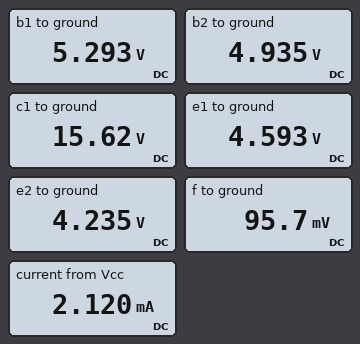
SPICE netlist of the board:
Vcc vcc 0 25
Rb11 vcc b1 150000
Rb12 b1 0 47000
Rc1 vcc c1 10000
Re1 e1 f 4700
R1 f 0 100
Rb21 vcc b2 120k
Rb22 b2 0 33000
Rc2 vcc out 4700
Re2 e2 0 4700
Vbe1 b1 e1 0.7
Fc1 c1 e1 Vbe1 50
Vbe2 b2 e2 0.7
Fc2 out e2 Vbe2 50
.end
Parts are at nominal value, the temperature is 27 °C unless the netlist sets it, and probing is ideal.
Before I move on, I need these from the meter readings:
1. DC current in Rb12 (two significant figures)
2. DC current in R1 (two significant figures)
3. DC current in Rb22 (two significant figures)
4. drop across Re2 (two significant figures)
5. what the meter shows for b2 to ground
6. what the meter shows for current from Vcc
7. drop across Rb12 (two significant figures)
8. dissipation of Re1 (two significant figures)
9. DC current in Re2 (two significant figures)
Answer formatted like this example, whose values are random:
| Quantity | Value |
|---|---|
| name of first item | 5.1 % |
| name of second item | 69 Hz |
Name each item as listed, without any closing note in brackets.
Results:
| Quantity | Value |
|---|---|
| DC current in Rb12 | 110 µA |
| DC current in R1 | 960 µA |
| DC current in Rb22 | 150 µA |
| drop across Re2 | 4.2 V |
| what the meter shows for b2 to ground | 4.935 V |
| what the meter shows for current from Vcc | 2.120 mA |
| drop across Rb12 | 5.3 V |
| dissipation of Re1 | 4.3 mW |
| DC current in Re2 | 900 µA |
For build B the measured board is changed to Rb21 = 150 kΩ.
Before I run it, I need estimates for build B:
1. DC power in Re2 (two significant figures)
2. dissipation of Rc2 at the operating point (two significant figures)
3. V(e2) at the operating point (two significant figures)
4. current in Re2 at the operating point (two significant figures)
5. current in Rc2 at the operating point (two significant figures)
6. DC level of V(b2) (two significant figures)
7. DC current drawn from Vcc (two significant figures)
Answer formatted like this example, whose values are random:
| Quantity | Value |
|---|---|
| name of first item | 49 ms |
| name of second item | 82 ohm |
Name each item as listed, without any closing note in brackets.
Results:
| Quantity | Value |
|---|---|
| DC power in Re2 | 2.5 mW |
| dissipation of Rc2 at the operating point | 2.4 mW |
| V(e2) at the operating point | 3.4 V |
| current in Re2 at the operating point | 730 µA |
| current in Rc2 at the operating point | 710 µA |
| DC level of V(b2) | 4.1 V |
| DC current drawn from Vcc | 1.9 mA |
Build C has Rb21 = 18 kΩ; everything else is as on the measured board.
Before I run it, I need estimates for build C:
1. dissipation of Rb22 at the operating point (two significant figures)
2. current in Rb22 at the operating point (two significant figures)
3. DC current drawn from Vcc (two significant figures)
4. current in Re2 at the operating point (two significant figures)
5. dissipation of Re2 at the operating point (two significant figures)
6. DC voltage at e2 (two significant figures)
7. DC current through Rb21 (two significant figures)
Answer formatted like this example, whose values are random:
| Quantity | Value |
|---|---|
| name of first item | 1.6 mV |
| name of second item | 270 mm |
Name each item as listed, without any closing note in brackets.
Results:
| Quantity | Value |
|---|---|
| dissipation of Rb22 at the operating point | 7.2 mW |
| current in Rb22 at the operating point | 470 µA |
| DC current drawn from Vcc | 4.7 mA |
| current in Re2 at the operating point | 3.1 mA |
| dissipation of Re2 at the operating point | 46 mW |
| DC voltage at e2 | 15 V |
| DC current through Rb21 | 530 µA |
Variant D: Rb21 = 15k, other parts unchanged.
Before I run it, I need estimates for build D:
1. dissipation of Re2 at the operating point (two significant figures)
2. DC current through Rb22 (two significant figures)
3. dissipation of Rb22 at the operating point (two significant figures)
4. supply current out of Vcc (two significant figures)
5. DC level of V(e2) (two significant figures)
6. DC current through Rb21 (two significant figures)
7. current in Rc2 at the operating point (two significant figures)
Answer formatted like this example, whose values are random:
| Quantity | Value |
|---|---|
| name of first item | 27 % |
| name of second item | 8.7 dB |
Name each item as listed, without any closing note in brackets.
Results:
| Quantity | Value |
|---|---|
| dissipation of Re2 at the operating point | 53 mW |
| DC current through Rb22 | 500 µA |
| dissipation of Rb22 at the operating point | 8.3 mW |
| supply current out of Vcc | 4.9 mA |
| DC level of V(e2) | 16 V |
| DC current through Rb21 | 570 µA |
| current in Rc2 at the operating point | 3.3 mA |
